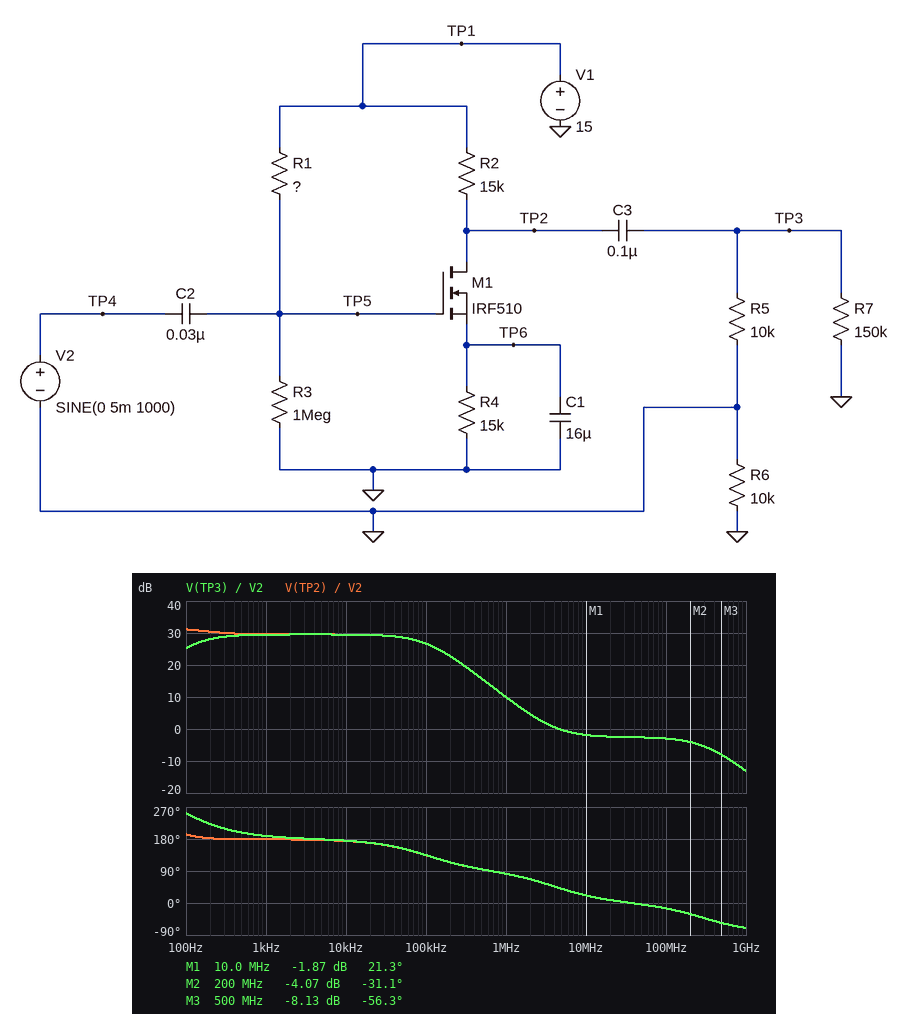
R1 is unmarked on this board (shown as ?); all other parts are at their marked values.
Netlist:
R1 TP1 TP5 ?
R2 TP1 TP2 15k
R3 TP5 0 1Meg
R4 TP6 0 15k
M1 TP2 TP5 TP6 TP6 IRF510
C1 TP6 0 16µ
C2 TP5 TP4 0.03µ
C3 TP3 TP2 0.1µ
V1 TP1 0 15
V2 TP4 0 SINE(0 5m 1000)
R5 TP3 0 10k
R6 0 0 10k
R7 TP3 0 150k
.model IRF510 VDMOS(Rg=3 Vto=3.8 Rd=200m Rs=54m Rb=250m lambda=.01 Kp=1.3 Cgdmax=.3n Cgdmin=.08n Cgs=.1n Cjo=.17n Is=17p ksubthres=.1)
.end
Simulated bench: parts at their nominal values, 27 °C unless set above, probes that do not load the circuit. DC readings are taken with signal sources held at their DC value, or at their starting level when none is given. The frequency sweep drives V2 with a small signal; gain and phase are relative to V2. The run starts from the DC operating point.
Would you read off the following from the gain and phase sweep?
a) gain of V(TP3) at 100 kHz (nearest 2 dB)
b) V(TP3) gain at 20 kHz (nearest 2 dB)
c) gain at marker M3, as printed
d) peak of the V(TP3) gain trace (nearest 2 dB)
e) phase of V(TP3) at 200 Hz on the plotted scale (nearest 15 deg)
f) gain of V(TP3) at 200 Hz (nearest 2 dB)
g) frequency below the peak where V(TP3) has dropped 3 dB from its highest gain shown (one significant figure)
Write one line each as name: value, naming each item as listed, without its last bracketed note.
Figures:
gain of V(TP3) at 100 kHz: 26 dB
V(TP3) gain at 20 kHz: 30 dB
gain at marker M3, as printed: -8.13 dB
peak of the V(TP3) gain trace: 30 dB
phase of V(TP3) at 200 Hz on the plotted scale: 225 deg
gain of V(TP3) at 200 Hz: 28 dB
frequency below the peak where V(TP3) has dropped 3 dB from its highest gain shown: 100 Hz
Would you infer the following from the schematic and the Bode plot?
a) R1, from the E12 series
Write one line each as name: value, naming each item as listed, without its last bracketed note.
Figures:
R1, from the E12 series: 470 kΩ
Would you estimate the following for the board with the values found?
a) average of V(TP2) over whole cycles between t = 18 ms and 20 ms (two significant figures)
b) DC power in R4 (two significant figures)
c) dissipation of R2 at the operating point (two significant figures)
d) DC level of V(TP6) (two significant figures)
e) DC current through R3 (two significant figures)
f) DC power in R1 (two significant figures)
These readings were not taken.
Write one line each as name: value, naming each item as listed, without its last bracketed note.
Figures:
average of V(TP2) over whole cycles between t = 18 ms and 20 ms: 8.5 V
DC power in R4: 2.8 mW
dissipation of R2 at the operating point: 2.8 mW
DC level of V(TP6): 6.5 V
DC current through R3: 10 µA
DC power in R1: 49 µW
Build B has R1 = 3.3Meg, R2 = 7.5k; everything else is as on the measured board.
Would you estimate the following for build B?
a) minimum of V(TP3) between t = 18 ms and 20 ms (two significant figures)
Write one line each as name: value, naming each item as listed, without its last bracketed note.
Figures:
minimum of V(TP3) between t = 18 ms and 20 ms: -1.7 mV
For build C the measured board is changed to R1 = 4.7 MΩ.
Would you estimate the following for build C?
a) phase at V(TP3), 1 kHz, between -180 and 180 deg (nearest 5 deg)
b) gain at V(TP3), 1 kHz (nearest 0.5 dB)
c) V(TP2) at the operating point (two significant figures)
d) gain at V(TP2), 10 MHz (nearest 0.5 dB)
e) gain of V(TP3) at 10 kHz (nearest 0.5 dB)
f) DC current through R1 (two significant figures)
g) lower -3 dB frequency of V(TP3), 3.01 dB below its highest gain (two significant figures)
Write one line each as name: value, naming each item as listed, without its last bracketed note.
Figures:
phase at V(TP3), 1 kHz, between -180 and 180 deg: 95 deg
gain at V(TP3), 1 kHz: -50.0 dB
V(TP2) at the operating point: 15 V
gain at V(TP2), 10 MHz: -3.0 dB
gain of V(TP3) at 10 kHz: -30.0 dB
DC current through R1: 2.6 µA
lower -3 dB frequency of V(TP3), 3.01 dB below its highest gain: 220 kHz
